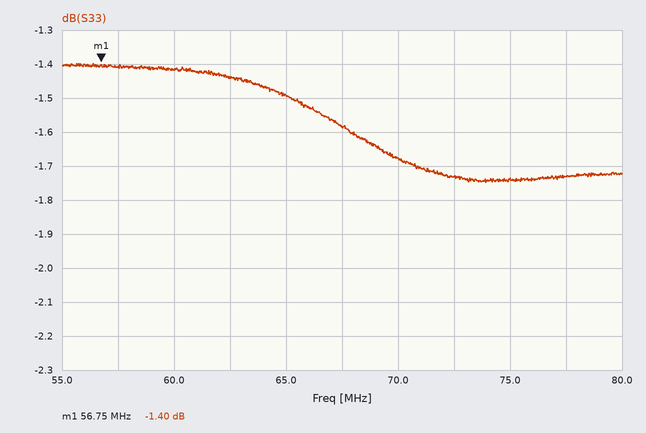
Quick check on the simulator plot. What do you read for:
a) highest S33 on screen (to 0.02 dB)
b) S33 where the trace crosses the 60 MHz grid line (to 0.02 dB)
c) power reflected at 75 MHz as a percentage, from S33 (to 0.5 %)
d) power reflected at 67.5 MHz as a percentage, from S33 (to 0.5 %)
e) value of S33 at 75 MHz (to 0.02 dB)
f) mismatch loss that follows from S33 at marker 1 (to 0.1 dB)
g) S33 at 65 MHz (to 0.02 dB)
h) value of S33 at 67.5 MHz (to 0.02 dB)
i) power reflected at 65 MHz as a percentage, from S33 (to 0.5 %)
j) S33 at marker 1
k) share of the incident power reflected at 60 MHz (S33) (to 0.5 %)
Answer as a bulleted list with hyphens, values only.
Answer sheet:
- -1.40 dB
- -1.42 dB
- 67.0 %
- 69.5 %
- -1.74 dB
- 5.6 dB
- -1.50 dB
- -1.58 dB
- 71.0 %
- -1.40 dB
- 72.0 %
